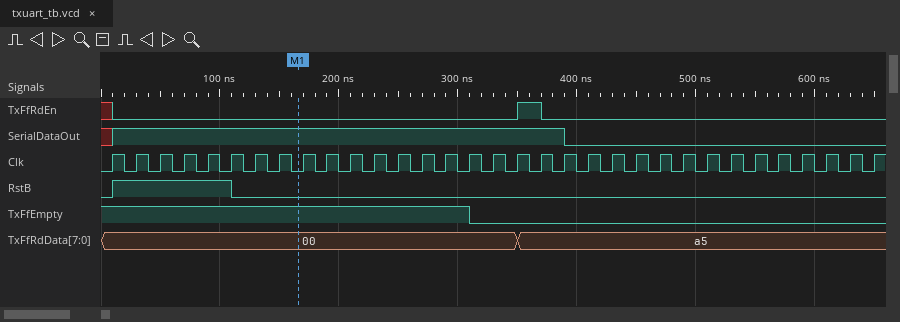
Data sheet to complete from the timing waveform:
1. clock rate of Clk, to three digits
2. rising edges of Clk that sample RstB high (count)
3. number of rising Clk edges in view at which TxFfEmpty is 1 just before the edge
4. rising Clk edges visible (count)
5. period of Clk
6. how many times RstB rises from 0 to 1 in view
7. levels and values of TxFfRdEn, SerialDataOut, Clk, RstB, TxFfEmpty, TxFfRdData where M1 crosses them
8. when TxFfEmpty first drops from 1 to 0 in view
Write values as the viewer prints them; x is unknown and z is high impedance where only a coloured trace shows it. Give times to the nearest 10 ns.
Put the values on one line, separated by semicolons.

50.0 MHz; 5; 16; 33; 20 ns; 1; TxFfRdEn=0, SerialDataOut=1, Clk=0, RstB=0, TxFfEmpty=1, TxFfRdData=00; 310 ns
